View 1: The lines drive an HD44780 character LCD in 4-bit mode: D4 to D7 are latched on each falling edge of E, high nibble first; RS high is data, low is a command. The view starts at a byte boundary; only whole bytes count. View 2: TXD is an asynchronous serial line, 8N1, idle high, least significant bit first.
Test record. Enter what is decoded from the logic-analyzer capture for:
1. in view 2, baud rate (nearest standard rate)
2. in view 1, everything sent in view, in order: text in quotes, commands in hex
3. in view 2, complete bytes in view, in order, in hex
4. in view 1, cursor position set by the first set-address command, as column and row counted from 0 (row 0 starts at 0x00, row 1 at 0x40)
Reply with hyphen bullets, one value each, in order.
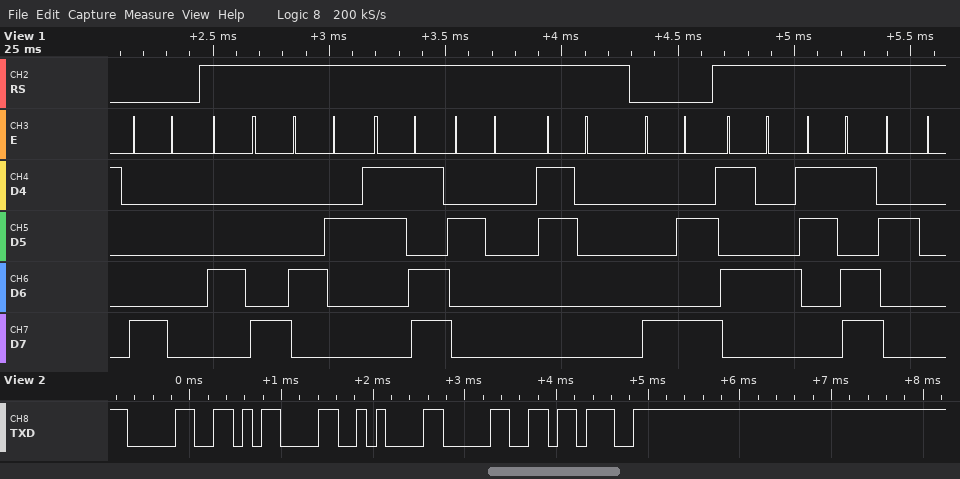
- 9600 baud
- 0x80 "HB= 0" 0x8A "T= "
- 0x30 0x0D 0x0A 0x30 0x3B
- column 0, row 0
